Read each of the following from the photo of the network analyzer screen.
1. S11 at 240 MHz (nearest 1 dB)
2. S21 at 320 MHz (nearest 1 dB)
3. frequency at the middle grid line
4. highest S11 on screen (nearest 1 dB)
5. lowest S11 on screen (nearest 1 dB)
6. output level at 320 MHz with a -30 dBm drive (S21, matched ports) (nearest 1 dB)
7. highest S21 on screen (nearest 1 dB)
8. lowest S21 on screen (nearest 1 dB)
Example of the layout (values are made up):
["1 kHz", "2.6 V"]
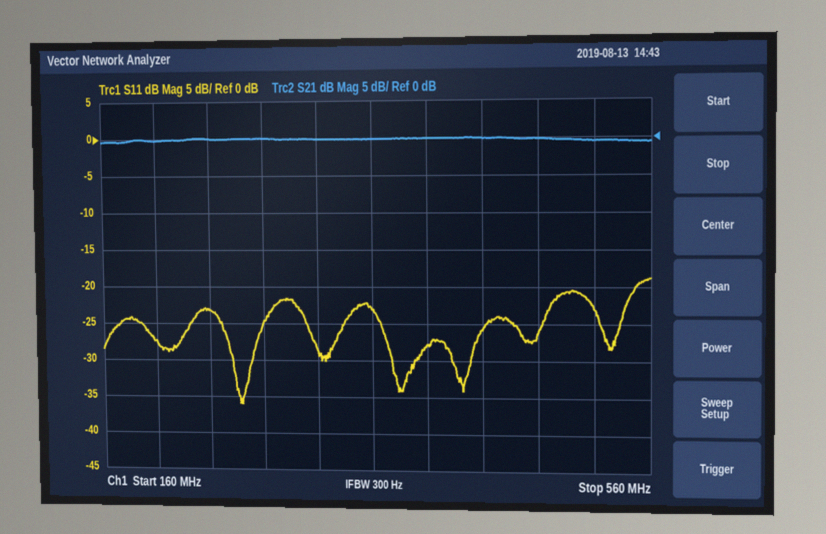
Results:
["-23 dB", "0 dB", "360 MHz", "-19 dB", "-36 dB", "-30 dBm", "0 dB", "-1 dB"]
